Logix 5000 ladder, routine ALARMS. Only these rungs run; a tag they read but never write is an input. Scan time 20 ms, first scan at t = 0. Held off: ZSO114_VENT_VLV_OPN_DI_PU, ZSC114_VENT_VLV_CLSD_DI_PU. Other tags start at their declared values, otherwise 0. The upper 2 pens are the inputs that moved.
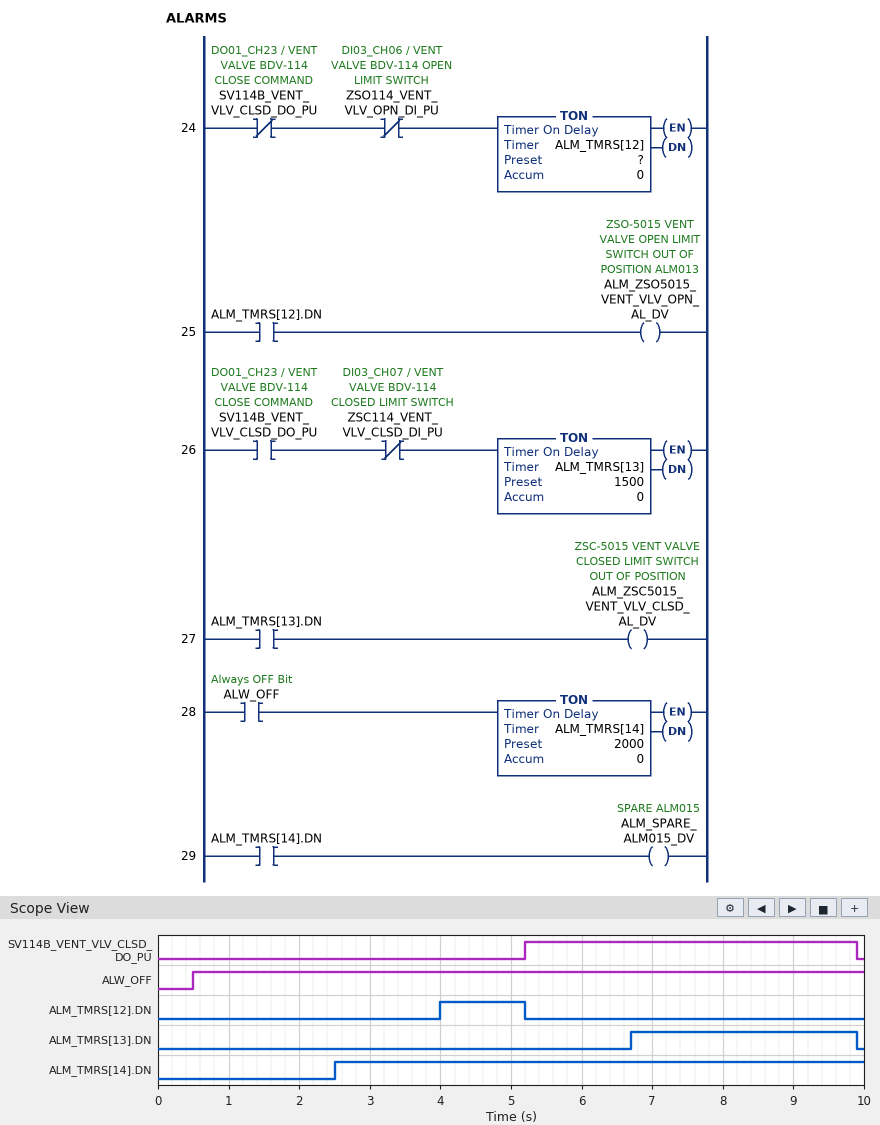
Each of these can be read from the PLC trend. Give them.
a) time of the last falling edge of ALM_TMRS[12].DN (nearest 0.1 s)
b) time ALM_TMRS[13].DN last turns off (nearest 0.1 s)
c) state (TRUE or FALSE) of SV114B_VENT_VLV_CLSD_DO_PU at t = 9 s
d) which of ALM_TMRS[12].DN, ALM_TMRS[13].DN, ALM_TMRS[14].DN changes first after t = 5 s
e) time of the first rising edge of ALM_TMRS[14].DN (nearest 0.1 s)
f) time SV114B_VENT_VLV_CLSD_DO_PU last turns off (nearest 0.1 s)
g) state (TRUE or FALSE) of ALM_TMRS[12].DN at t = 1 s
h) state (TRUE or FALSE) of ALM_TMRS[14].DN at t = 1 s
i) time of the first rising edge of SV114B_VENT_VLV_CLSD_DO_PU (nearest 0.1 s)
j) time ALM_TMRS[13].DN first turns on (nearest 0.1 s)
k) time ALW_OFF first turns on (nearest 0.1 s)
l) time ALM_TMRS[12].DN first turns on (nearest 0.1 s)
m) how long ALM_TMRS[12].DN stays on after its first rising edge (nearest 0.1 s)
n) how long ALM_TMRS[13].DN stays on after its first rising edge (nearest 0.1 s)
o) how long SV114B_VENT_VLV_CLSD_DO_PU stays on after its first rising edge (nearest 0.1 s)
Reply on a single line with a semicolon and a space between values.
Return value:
5.2 s; 9.9 s; TRUE; ALM_TMRS[12].DN; 2.5 s; 9.9 s; FALSE; FALSE; 5.2 s; 6.7 s; 0.5 s; 4.0 s; 1.2 s; 3.2 s; 4.7 s
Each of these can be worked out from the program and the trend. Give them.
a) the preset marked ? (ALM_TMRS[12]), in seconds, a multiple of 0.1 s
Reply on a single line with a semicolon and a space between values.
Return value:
4.0 s
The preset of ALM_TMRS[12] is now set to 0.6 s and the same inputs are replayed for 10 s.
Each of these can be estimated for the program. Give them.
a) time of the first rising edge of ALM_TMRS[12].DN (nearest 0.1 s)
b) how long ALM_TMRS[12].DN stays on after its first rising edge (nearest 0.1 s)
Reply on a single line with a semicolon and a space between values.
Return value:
0.6 s; 4.6 s
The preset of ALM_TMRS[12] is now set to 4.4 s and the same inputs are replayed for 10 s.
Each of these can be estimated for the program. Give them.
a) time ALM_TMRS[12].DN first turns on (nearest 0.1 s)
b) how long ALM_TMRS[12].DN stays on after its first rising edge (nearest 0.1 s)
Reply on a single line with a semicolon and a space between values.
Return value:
4.4 s; 0.8 s
